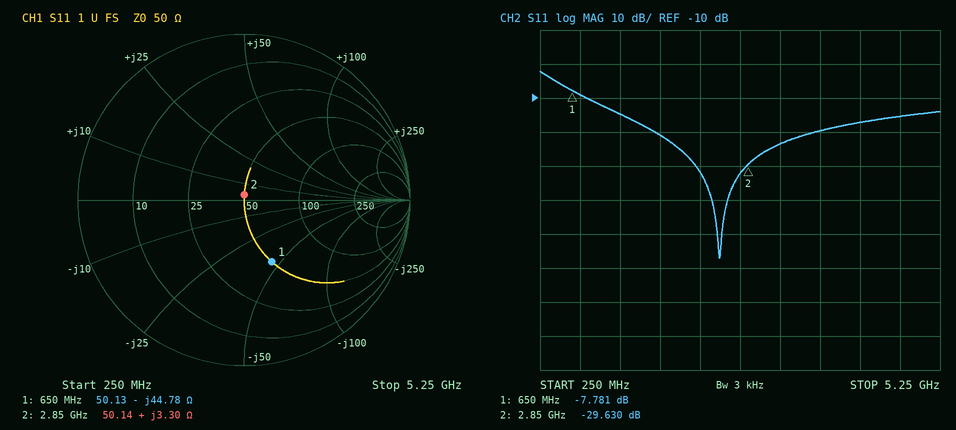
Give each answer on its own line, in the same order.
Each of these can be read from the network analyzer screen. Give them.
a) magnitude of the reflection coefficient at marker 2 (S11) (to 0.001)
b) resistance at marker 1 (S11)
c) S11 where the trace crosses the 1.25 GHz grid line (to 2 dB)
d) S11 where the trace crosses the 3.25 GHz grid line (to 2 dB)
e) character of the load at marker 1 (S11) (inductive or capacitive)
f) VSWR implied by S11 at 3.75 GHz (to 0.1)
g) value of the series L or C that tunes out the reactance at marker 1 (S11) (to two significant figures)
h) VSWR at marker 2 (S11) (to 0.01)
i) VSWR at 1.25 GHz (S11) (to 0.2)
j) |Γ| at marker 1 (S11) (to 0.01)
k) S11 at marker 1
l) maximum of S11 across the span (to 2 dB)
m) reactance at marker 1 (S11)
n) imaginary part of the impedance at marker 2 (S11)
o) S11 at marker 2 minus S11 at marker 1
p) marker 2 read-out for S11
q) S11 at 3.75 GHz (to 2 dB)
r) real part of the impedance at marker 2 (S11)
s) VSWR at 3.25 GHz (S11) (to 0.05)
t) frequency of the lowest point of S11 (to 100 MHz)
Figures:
0.033
50.13 Ω
-14 dB
-24 dB
capacitive
1.2
11 nH
1.07
1.4
0.41
-7.781 dB
-2 dB
-44.78 Ω
+3.30 Ω
-21.849 dB
-29.630 dB
-20 dB
50.14 Ω
1.15
2.5 GHz
